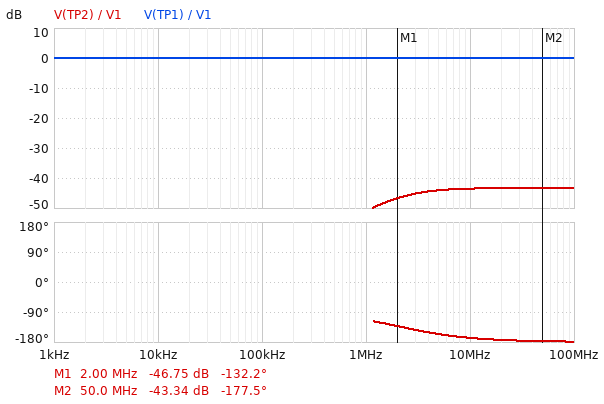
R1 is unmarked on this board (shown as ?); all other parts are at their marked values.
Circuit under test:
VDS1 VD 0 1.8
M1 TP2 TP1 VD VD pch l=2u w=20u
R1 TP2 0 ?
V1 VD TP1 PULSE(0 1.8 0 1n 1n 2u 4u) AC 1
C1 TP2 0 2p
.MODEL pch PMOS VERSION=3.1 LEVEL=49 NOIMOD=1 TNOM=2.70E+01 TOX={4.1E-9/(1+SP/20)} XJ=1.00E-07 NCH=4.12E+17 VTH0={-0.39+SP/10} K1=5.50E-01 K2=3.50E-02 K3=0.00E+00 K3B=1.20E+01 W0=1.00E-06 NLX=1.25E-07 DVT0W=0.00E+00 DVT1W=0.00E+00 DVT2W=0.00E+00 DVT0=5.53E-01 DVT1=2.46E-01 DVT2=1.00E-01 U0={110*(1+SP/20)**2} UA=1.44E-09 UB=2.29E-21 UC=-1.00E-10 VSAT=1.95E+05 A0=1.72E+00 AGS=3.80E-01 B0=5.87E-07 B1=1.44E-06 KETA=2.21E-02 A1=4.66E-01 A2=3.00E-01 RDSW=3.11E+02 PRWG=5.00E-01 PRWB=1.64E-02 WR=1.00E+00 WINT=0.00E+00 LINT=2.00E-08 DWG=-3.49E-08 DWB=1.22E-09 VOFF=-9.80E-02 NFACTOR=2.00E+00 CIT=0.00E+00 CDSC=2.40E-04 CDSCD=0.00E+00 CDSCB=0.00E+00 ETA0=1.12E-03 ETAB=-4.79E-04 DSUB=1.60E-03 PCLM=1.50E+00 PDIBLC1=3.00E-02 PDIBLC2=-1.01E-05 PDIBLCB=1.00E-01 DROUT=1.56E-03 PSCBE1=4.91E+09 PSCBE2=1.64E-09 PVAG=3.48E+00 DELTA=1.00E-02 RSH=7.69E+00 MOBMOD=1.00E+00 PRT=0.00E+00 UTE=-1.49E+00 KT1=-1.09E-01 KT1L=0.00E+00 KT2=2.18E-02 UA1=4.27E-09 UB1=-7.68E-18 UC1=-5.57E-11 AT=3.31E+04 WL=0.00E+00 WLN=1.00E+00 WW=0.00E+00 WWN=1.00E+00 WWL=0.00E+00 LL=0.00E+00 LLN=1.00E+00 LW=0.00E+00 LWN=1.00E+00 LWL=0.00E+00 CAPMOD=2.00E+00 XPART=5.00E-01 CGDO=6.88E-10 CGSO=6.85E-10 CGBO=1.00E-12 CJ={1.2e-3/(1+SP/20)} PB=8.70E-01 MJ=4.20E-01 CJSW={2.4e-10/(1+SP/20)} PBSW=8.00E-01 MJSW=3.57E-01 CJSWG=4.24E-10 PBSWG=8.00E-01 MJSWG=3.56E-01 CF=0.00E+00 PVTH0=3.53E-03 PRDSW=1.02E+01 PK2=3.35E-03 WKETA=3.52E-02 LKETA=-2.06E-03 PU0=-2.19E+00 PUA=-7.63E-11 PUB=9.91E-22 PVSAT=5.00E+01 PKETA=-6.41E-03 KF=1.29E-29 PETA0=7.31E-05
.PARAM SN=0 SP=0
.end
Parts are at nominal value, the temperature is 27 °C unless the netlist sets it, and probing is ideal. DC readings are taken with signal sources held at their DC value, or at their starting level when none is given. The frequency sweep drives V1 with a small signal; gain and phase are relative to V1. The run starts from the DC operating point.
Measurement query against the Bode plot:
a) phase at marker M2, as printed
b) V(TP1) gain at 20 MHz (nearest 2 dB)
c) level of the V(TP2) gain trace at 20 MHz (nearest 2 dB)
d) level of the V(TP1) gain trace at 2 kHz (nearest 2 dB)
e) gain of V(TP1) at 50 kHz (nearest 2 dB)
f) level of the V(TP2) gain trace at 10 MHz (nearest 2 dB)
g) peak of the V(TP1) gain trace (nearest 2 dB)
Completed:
-177.5 deg
0 dB
-44 dB
0 dB
0 dB
-44 dB
0 dB
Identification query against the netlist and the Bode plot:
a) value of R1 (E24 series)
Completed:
36 kΩ
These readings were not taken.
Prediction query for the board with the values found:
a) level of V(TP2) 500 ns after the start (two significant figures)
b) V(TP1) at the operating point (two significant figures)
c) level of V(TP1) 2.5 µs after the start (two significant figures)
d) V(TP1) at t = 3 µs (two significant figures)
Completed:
1.7 V
1.8 V
1.8 V
1.8 V
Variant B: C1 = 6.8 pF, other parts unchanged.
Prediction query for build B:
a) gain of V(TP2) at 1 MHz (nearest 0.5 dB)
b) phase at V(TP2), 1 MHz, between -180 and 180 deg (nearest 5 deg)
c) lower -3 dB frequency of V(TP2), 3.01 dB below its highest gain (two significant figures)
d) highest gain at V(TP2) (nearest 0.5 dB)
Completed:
-55.5 dB
-145 deg
650 kHz
-54.0 dB
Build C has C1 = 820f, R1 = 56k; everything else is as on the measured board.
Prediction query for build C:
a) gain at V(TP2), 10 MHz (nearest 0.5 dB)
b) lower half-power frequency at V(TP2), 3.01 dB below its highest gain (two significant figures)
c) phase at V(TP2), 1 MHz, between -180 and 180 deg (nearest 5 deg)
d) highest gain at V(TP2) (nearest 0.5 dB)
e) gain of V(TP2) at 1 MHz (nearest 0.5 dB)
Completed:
-36.0 dB
3.4 MHz
-105 deg
-35.5 dB
-46.5 dB
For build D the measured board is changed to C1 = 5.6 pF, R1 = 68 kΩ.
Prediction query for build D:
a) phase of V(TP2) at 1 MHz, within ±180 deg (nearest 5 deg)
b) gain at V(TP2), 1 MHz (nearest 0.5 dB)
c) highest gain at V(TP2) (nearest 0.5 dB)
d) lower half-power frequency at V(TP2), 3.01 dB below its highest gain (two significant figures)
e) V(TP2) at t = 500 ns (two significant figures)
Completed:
-155 deg
-53.0 dB
-52.0 dB
420 kHz
1.8 V
